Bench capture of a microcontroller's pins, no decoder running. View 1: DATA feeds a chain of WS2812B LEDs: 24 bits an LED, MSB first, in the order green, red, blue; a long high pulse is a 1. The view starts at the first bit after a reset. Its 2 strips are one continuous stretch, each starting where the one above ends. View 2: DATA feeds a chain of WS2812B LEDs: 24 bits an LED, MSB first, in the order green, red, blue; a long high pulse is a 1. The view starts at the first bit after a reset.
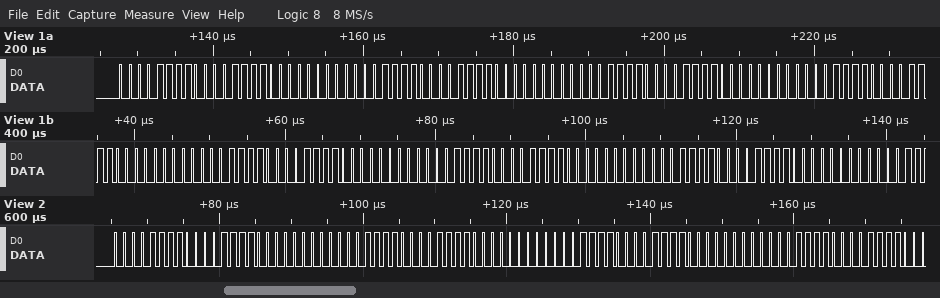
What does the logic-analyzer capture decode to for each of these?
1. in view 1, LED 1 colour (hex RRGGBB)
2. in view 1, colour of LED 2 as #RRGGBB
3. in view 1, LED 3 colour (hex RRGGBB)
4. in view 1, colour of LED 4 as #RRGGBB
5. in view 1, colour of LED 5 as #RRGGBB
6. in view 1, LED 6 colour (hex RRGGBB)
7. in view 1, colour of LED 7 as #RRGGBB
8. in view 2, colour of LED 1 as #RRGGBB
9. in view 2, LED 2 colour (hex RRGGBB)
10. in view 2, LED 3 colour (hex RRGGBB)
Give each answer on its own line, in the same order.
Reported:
#0F0F00
#0F0F00
#0F0F00
#0F0F00
#0F0F00
#0F0F00
#0F0F00
#0F0F00
#0F0F00
#0F0F00
